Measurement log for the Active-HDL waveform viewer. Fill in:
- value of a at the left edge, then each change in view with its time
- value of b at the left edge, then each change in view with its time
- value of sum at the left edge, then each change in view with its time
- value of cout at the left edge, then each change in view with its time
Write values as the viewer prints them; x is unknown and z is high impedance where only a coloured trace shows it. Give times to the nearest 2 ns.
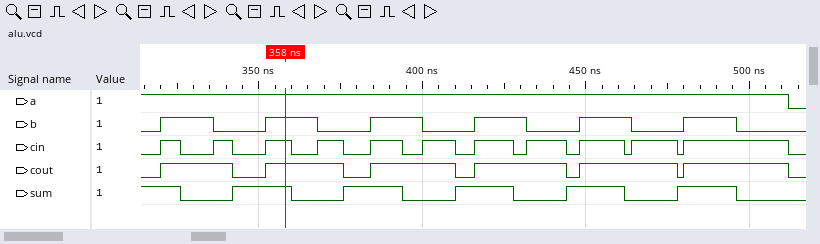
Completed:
1, 0 at 512 ns
0, 1 at 320 ns, 0 at 336 ns, 1 at 352 ns, 0 at 368 ns, 1 at 384 ns, 0 at 400 ns, 1 at 416 ns, 0 at 432 ns, 1 at 448 ns, 0 at 464 ns, 1 at 480 ns, 0 at 496 ns
1, 0 at 326 ns, 1 at 342 ns, 0 at 360 ns, 1 at 376 ns, 0 at 394 ns, 1 at 410 ns, 0 at 428 ns, 1 at 444 ns, 0 at 462 ns, 1 at 478 ns, 0 at 496 ns
0, 1 at 320 ns, 0 at 342 ns, 1 at 352 ns, 0 at 376 ns, 1 at 384 ns, 0 at 410 ns, 1 at 416 ns, 0 at 444 ns, 1 at 448 ns, 0 at 478 ns, 1 at 480 ns, 0 at 512 ns
